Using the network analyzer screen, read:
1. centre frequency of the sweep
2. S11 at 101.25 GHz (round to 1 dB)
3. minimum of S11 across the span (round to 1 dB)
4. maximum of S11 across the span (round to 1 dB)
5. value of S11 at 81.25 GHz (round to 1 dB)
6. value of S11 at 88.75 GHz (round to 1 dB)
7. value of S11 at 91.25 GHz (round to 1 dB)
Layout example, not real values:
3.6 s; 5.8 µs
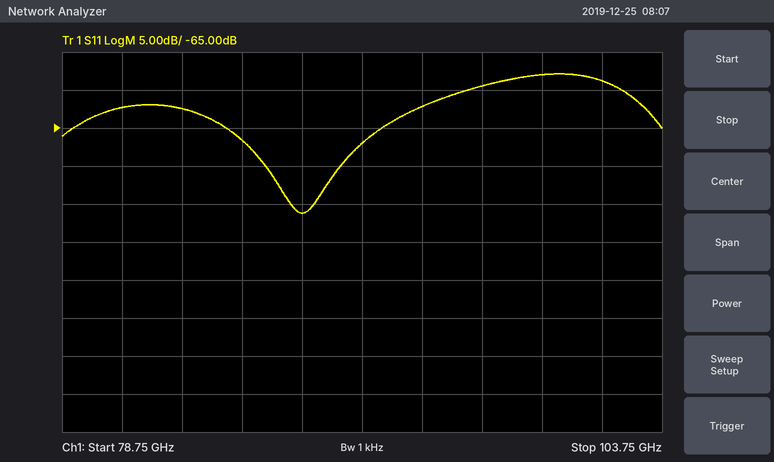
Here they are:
91.25 GHz; -59 dB; -76 dB; -58 dB; -62 dB; -76 dB; -67 dB
